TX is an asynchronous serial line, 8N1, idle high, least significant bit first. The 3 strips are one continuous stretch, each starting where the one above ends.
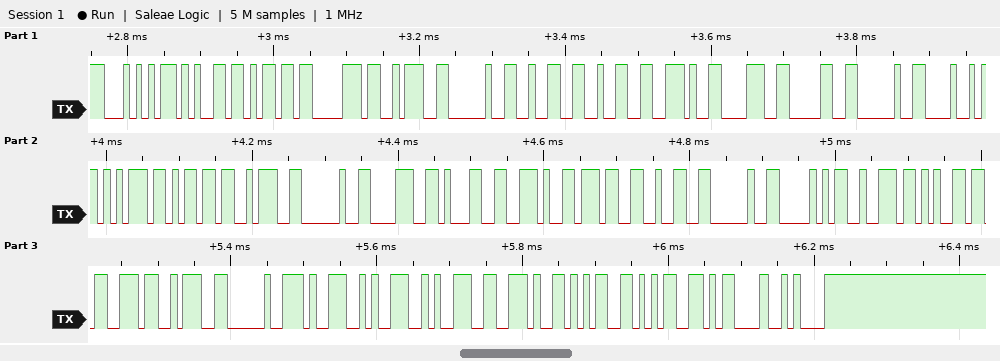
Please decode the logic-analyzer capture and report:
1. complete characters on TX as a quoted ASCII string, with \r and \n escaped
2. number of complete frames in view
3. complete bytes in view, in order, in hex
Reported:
"Temp: 22.80 Hum: 81.72 Pres: 999.55\r\n"
37
0x54 0x65 0x6D 0x70 0x3A 0x20 0x32 0x32 0x2E 0x38 0x30 0x20 0x48 0x75 0x6D 0x3A 0x20 0x38 0x31 0x2E 0x37 0x32 0x20 0x50 0x72 0x65 0x73 0x3A 0x20 0x39 0x39 0x39 0x2E 0x35 0x35 0x0D 0x0A
